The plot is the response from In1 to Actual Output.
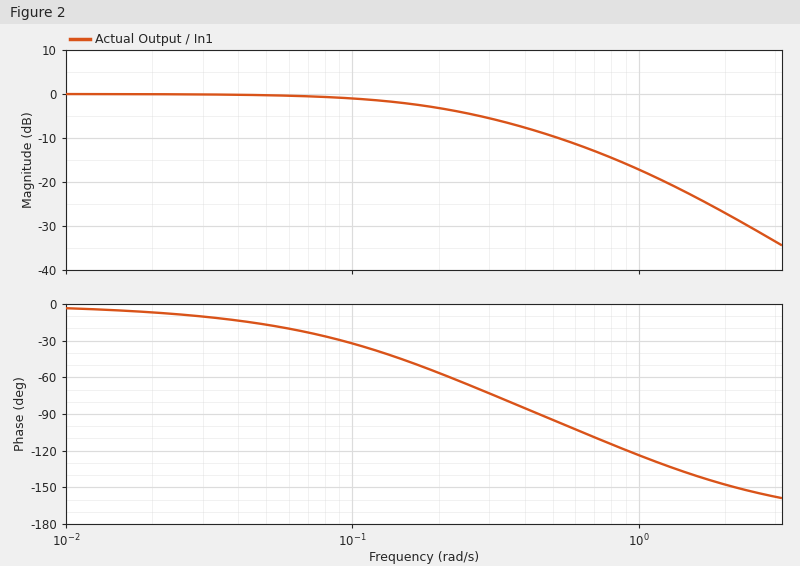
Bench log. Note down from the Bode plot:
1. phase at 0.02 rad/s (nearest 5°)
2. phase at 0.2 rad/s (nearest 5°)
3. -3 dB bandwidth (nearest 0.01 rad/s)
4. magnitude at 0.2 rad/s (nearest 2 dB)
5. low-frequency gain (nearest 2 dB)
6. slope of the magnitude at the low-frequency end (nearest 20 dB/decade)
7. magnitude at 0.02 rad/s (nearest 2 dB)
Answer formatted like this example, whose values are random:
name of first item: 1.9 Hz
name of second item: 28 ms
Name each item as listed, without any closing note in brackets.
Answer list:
phase at 0.02 rad/s: -5°
phase at 0.2 rad/s: -55°
-3 dB bandwidth: 0.19 rad/s
magnitude at 0.2 rad/s: -4 dB
low-frequency gain: 0 dB
slope of the magnitude at the low-frequency end: 0 dB/decade
magnitude at 0.02 rad/s: 0 dB
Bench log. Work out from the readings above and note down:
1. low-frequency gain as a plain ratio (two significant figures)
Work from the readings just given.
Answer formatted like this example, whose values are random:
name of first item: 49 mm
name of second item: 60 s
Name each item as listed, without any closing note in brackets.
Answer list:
low-frequency gain as a plain ratio: 1.0
